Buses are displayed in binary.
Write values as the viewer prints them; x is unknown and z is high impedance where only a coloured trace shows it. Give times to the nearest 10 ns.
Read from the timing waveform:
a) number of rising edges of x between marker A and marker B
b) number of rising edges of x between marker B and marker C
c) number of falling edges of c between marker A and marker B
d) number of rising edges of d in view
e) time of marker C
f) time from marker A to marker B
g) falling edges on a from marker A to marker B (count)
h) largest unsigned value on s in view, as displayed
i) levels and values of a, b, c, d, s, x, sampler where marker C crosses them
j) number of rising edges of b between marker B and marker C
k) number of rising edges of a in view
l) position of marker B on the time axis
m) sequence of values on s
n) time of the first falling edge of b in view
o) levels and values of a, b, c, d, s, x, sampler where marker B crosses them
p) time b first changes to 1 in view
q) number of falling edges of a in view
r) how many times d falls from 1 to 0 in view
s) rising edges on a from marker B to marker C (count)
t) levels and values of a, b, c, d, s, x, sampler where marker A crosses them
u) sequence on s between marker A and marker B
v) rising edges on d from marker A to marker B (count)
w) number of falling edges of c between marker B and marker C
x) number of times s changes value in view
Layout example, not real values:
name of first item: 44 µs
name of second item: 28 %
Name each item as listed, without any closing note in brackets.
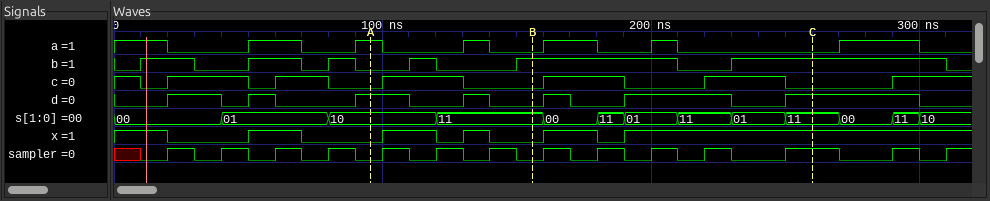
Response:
number of rising edges of x between marker A and marker B: 2
number of rising edges of x between marker B and marker C: 2
number of falling edges of c between marker A and marker B: 1
number of rising edges of d in view: 7
time of marker C: 260 ns
time from marker A to marker B: 60 ns
falling edges on a from marker A to marker B: 2
largest unsigned value on s in view, as displayed: 11
levels and values of a, b, c, d, s, x, sampler where marker C crosses them: a=0, b=1, c=0, d=1, s=11, x=1, sampler=1
number of rising edges of b between marker B and marker C: 1
number of rising edges of a in view: 6
position of marker B on the time axis: 160 ns
sequence of values on s: 00, 01, 10, 11, 00, 11, 01, 11, 01, 11, 00, 11, 10
time of the first falling edge of b in view: 30 ns
levels and values of a, b, c, d, s, x, sampler where marker B crosses them: a=0, b=1, c=0, d=0, s=11, x=0, sampler=0
time b first changes to 1 in view: 10 ns
number of falling edges of a in view: 7
how many times d falls from 1 to 0 in view: 7
rising edges on a from marker B to marker C: 2
levels and values of a, b, c, d, s, x, sampler where marker A crosses them: a=1, b=0, c=0, d=1, s=10, x=0, sampler=0
sequence on s between marker A and marker B: 10, 11
rising edges on d from marker A to marker B: 1
number of falling edges of c between marker B and marker C: 2
number of times s changes value in view: 12
